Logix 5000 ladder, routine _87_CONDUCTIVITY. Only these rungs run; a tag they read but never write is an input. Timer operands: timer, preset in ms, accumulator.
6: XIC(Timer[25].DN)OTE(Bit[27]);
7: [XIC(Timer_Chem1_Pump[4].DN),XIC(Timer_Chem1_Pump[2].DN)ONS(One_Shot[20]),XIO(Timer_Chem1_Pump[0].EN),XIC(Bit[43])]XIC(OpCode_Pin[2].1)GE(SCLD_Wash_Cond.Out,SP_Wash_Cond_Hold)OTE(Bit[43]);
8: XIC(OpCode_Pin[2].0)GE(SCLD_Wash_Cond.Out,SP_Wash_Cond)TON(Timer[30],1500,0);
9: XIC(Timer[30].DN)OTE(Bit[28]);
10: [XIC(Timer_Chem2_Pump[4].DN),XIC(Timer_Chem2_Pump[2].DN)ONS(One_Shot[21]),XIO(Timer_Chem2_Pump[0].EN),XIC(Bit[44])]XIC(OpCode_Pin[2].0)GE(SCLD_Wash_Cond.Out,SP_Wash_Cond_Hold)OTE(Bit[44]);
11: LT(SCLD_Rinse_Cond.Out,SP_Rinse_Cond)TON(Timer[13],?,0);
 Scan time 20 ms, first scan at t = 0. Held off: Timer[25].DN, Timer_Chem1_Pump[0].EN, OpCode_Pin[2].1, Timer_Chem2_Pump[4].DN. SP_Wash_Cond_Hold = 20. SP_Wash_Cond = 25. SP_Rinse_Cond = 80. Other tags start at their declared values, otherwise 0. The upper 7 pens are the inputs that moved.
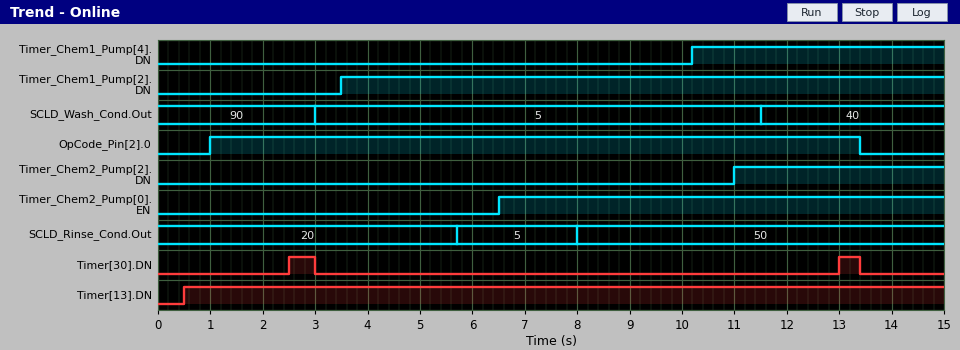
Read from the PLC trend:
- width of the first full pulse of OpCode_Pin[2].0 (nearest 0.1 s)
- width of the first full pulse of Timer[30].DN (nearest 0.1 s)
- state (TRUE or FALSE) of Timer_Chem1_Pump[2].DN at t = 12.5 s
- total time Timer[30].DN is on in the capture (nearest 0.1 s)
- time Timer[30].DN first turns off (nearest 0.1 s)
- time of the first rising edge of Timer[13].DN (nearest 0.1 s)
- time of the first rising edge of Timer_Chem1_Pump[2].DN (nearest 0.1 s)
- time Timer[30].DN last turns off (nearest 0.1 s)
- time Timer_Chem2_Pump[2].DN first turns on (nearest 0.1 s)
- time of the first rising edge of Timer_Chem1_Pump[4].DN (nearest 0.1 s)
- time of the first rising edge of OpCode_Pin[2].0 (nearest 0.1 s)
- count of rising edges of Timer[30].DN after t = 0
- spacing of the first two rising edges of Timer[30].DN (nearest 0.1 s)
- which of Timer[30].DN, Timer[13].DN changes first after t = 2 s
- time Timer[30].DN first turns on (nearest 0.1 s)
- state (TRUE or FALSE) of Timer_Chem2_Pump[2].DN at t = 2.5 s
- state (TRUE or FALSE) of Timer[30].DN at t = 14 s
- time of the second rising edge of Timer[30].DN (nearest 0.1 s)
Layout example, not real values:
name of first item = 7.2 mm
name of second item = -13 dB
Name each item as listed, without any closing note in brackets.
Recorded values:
width of the first full pulse of OpCode_Pin[2].0 = 12.4 s
width of the first full pulse of Timer[30].DN = 0.5 s
state (TRUE or FALSE) of Timer_Chem1_Pump[2].DN at t = 12.5 s = TRUE
total time Timer[30].DN is on in the capture = 0.9 s
time Timer[30].DN first turns off = 3.0 s
time of the first rising edge of Timer[13].DN = 0.5 s
time of the first rising edge of Timer_Chem1_Pump[2].DN = 3.5 s
time Timer[30].DN last turns off = 13.4 s
time Timer_Chem2_Pump[2].DN first turns on = 11.0 s
time of the first rising edge of Timer_Chem1_Pump[4].DN = 10.2 s
time of the first rising edge of OpCode_Pin[2].0 = 1.0 s
count of rising edges of Timer[30].DN after t = 0 = 2
spacing of the first two rising edges of Timer[30].DN = 10.5 s
which of Timer[30].DN, Timer[13].DN changes first after t = 2 s = Timer[30].DN
time Timer[30].DN first turns on = 2.5 s
state (TRUE or FALSE) of Timer_Chem2_Pump[2].DN at t = 2.5 s = FALSE
state (TRUE or FALSE) of Timer[30].DN at t = 14 s = FALSE
time of the second rising edge of Timer[30].DN = 13.0 s
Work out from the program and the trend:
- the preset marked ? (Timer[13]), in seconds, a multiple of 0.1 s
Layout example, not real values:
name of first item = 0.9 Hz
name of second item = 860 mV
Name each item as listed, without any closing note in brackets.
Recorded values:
the preset marked ? (Timer[13]), in seconds, a multiple of 0.1 s = 0.5 s
